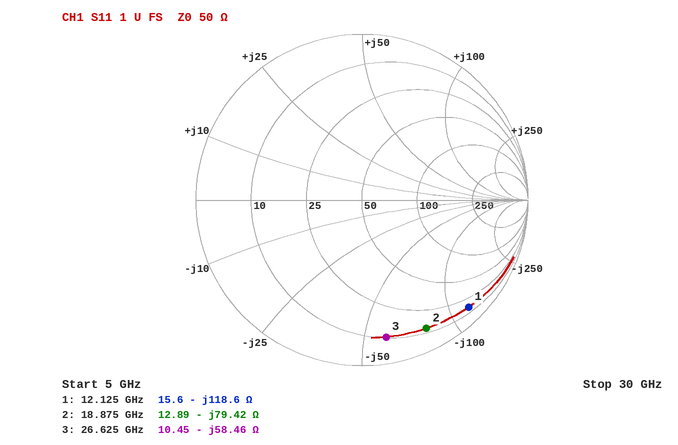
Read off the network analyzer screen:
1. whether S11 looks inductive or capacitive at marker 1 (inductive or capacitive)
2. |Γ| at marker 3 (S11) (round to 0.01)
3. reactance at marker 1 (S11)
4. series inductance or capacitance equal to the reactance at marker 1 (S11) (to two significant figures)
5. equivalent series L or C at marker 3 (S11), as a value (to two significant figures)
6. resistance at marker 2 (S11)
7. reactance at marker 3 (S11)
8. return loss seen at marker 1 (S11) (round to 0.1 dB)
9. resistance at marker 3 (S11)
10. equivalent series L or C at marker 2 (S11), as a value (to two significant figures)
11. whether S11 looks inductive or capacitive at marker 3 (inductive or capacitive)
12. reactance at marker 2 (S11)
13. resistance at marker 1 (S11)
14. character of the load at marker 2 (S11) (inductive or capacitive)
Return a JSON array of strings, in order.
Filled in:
["capacitive", "0.84", "-118.6 Ω", "110 fF", "100 fF", "12.89 Ω", "-58.46 Ω", "0.8 dB", "10.45 Ω", "110 fF", "capacitive", "-79.42 Ω", "15.6 Ω", "capacitive"]
